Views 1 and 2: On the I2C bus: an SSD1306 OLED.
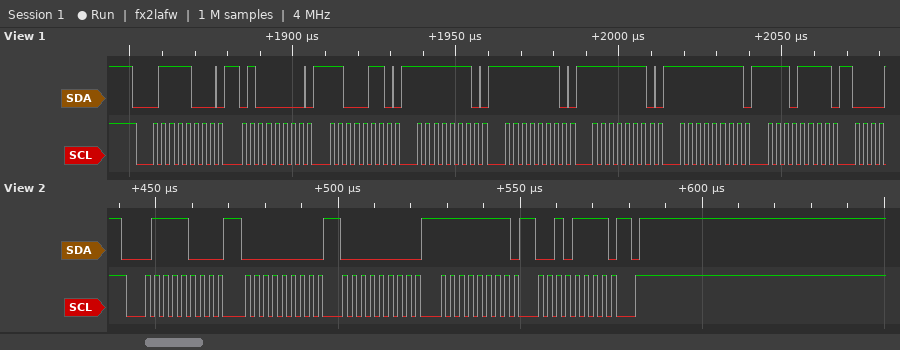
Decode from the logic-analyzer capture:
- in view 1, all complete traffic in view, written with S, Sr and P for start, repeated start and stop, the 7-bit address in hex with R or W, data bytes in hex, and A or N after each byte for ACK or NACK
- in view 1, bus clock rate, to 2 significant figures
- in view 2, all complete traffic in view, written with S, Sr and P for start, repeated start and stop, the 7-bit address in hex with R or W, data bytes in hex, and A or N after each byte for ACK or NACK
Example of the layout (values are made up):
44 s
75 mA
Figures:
S 3CW A 40 A C6 A FE A FE A FE A FF A EF A
400 kHz
S 3CW A 00 A 00 A FF A 2F A P
